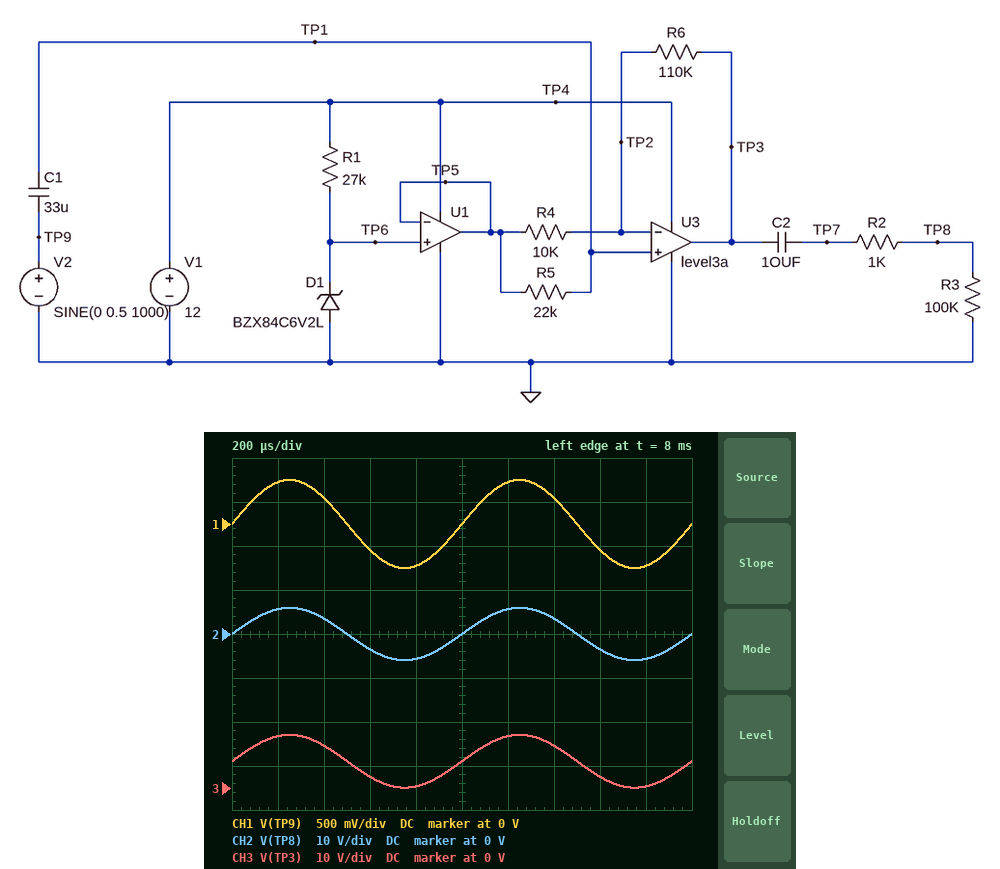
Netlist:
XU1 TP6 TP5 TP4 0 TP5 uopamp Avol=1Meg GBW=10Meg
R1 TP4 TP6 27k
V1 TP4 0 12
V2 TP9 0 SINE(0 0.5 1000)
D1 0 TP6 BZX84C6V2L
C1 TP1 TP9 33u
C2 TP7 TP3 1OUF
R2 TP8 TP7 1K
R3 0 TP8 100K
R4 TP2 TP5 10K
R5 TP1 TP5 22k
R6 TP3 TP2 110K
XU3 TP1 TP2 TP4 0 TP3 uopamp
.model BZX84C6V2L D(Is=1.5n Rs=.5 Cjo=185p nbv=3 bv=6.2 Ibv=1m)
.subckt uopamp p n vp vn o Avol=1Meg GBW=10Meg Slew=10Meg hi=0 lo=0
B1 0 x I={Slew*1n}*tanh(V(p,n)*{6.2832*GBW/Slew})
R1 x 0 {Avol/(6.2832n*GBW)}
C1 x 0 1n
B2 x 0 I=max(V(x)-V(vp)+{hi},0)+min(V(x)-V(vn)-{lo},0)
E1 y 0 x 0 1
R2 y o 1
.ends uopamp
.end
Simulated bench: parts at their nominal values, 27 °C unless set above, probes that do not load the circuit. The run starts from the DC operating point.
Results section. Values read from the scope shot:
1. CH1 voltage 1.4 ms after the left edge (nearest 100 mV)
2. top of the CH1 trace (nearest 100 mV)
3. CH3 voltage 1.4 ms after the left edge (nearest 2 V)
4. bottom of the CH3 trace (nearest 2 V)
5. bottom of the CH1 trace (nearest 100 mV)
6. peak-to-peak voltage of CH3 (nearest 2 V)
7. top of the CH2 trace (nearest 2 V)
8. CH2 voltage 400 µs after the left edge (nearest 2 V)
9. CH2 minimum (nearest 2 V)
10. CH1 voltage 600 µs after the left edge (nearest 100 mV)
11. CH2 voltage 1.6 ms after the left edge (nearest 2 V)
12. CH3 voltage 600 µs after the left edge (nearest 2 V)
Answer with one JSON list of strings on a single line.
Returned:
["300 mV", "500 mV", "10 V", "0 V", "-500 mV", "12 V", "6 V", "4 V", "-6 V", "-300 mV", "-4 V", "2 V"]
